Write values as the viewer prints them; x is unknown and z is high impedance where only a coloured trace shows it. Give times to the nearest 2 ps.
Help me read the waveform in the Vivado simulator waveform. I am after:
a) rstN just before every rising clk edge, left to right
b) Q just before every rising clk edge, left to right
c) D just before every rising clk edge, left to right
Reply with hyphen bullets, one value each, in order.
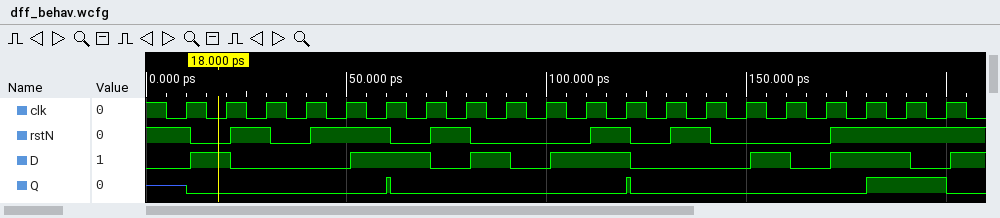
- 1 0 1 0 1 1 0 1 0 0 0 1 0 1 0 0 0 1 1 1
- z 0 0 0 0 0 0 0 0 0 0 0 0 0 0 0 0 0 1 1
- 0 1 0 0 0 1 1 0 1 0 1 1 0 0 0 1 0 1 1 0
